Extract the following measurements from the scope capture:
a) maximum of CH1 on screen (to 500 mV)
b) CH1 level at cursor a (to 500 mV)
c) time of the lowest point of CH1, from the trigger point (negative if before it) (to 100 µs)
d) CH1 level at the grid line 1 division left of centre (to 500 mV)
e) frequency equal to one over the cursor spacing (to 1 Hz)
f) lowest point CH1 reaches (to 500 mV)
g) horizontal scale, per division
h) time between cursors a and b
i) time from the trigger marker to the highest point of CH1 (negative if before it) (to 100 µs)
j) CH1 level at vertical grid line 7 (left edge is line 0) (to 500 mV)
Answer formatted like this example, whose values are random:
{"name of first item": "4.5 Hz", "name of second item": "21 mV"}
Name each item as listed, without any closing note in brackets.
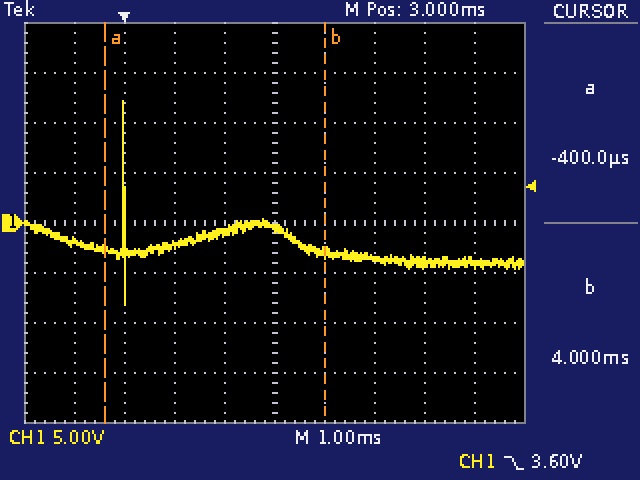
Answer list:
{"maximum of CH1 on screen": "12.0 V", "CH1 level at cursor a": "-2.5 V", "time of the lowest point of CH1, from the trigger point (negative if before it)": "0.0 ms", "CH1 level at the grid line 1 division left of centre": "-1.0 V", "frequency equal to one over the cursor spacing": "227 Hz", "lowest point CH1 reaches": "-8.0 V", "horizontal scale, per division": "1 ms", "time between cursors a and b": "4.4 ms", "time from the trigger marker to the highest point of CH1 (negative if before it)": "0.0 ms", "CH1 level at vertical grid line 7 (left edge is line 0)": "-3.5 V"}
